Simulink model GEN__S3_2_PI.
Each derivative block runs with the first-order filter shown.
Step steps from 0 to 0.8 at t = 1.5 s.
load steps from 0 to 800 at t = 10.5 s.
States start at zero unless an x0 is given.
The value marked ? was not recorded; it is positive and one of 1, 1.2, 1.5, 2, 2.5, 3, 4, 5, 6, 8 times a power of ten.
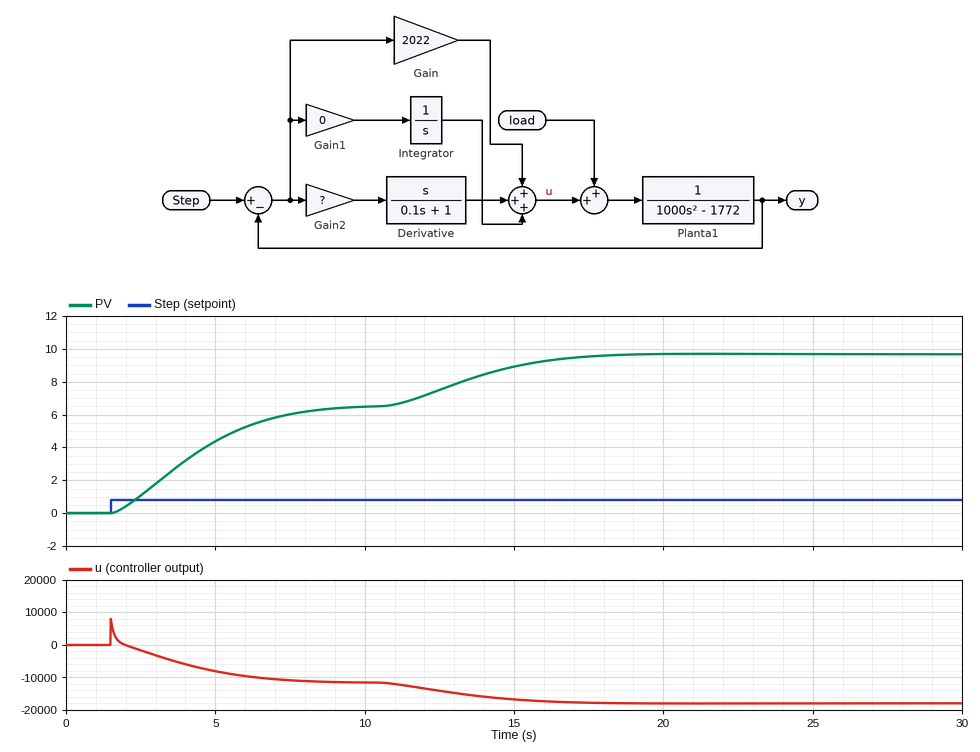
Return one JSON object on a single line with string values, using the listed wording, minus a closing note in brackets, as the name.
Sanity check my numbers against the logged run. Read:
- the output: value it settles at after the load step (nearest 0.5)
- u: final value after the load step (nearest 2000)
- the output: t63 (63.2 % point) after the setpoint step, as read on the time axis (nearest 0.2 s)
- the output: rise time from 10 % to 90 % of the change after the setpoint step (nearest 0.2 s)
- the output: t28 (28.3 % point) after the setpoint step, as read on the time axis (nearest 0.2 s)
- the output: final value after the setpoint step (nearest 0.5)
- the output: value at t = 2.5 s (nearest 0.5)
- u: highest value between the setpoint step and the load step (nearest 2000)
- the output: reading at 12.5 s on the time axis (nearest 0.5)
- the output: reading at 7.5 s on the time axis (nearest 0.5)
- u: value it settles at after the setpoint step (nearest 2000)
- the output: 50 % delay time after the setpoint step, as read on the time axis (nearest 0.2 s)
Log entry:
{"the output: value it settles at after the load step": "9.5", "u: final value after the load step": "-18000", "the output: t63 (63.2 % point) after the setpoint step, as read on the time axis": "4.8 s", "the output: rise time from 10 % to 90 % of the change after the setpoint step": "4.8 s", "the output: t28 (28.3 % point) after the setpoint step, as read on the time axis": "3.0 s", "the output: final value after the setpoint step": "6.5", "the output: value at t = 2.5 s": "1.0", "u: highest value between the setpoint step and the load step": "8000", "the output: reading at 12.5 s on the time axis": "7.5", "the output: reading at 7.5 s on the time axis": "6.0", "u: value it settles at after the setpoint step": "-12000", "the output: 50 % delay time after the setpoint step, as read on the time axis": "4.0 s"}
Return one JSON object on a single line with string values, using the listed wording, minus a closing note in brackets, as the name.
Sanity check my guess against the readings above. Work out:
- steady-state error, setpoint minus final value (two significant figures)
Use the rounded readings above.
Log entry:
{"steady-state error, setpoint minus final value": "-5.7"}
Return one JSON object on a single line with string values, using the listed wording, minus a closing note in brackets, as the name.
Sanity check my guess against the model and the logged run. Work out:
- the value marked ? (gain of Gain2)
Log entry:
{"the value marked ?": "800"}
